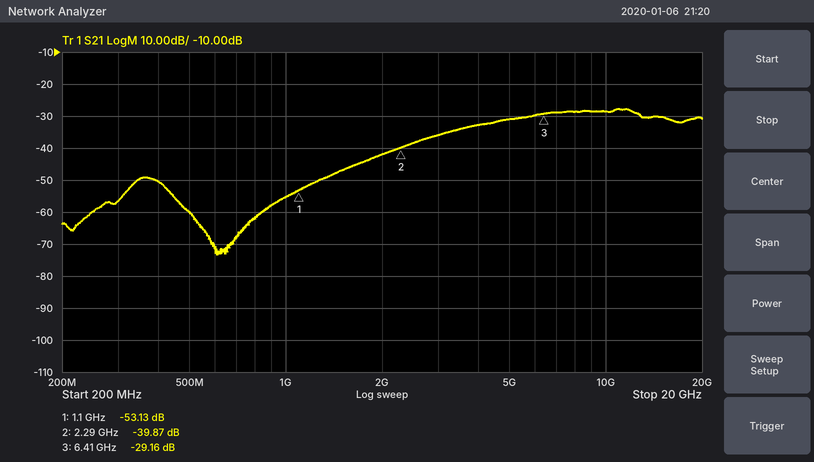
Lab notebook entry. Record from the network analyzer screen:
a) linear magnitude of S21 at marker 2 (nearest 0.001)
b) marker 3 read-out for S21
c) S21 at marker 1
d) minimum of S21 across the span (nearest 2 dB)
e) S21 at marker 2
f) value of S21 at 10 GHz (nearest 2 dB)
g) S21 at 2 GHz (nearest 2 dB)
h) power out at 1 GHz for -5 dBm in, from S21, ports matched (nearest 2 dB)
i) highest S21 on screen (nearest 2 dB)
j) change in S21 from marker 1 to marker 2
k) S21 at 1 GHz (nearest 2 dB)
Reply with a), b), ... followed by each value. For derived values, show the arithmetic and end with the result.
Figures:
a) 10^(-39.87/20) ≈ 0.010
b) -29.16 dB
c) -53.13 dB
d) -74 dB
e) -39.87 dB
f) -28 dB
g) -42 dB
h) -5 dBm + (-56 dB) = -60 dBm
i) -28 dB
j) -39.87 − (-53.13) = 13.26 dB
k) -56 dB
